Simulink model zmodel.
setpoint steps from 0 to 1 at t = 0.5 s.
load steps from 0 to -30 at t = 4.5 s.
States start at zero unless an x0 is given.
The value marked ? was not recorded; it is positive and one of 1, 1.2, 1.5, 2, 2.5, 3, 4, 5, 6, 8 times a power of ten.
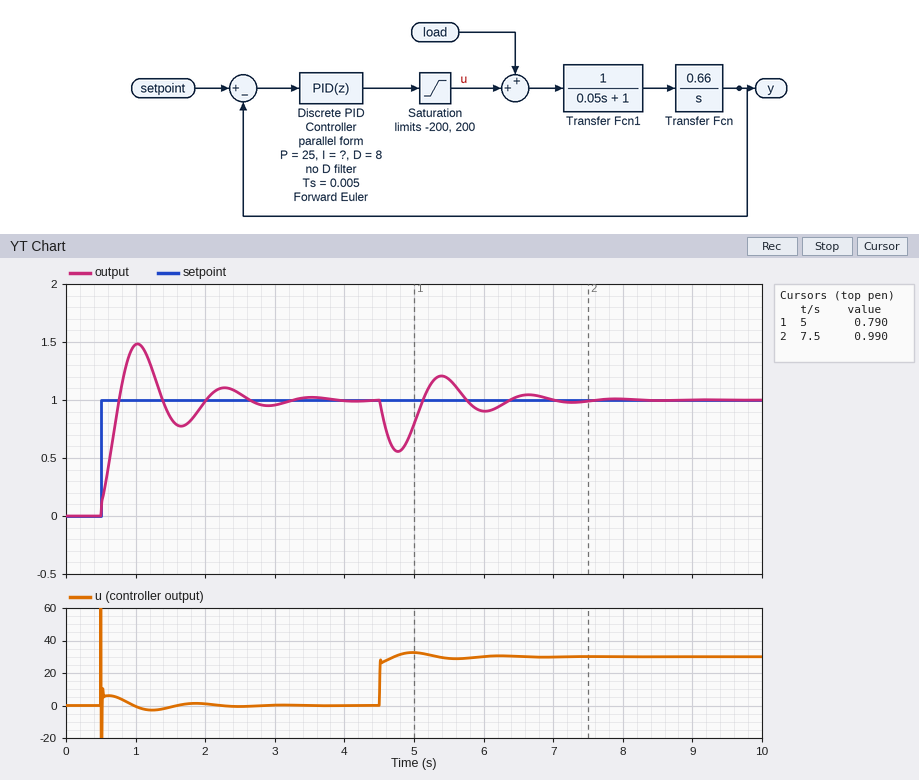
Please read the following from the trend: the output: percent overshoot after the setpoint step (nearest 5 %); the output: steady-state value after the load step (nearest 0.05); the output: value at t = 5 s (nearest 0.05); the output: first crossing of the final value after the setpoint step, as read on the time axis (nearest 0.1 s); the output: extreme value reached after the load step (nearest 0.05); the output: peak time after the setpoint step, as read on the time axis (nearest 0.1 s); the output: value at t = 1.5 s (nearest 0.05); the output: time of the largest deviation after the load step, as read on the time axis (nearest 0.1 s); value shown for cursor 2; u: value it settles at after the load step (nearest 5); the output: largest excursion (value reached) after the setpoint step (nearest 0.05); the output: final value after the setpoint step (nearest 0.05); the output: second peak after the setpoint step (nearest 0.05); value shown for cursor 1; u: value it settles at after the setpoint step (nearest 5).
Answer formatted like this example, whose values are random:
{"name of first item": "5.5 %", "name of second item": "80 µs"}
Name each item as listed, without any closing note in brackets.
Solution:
{"the output: percent overshoot after the setpoint step": "50 %", "the output: steady-state value after the load step": "1.00", "the output: value at t = 5 s": "0.80", "the output: first crossing of the final value after the setpoint step, as read on the time axis": "0.8 s", "the output: extreme value reached after the load step": "0.55", "the output: peak time after the setpoint step, as read on the time axis": "1.0 s", "the output: value at t = 1.5 s": "0.85", "the output: time of the largest deviation after the load step, as read on the time axis": "4.8 s", "value shown for cursor 2": "0.990", "u: value it settles at after the load step": "30", "the output: largest excursion (value reached) after the setpoint step": "1.50", "the output: final value after the setpoint step": "1.00", "the output: second peak after the setpoint step": "1.10", "value shown for cursor 1": "0.790", "u: value it settles at after the setpoint step": "0"}
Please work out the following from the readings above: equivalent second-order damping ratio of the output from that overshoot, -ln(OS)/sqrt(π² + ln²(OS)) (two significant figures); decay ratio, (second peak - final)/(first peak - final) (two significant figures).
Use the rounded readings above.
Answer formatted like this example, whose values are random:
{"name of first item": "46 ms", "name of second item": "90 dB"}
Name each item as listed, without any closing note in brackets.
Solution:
{"equivalent second-order damping ratio of the output from that overshoot, -ln(OS)/sqrt(π² + ln²(OS))": "0.22", "decay ratio, (second peak - final)/(first peak - final)": "0.20"}
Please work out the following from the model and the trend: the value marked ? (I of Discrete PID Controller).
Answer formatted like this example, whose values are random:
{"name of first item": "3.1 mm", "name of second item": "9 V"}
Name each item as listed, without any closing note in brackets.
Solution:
{"the value marked ?": "250"}
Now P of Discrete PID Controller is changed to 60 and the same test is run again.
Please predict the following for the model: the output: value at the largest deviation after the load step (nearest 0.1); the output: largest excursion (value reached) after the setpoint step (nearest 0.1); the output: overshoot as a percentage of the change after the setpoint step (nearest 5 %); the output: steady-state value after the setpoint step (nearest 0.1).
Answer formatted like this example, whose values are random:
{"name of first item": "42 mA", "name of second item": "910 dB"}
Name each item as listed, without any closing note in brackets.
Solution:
{"the output: value at the largest deviation after the load step": "0.7", "the output: largest excursion (value reached) after the setpoint step": "1.2", "the output: overshoot as a percentage of the change after the setpoint step": "25 %", "the output: steady-state value after the setpoint step": "1.0"}
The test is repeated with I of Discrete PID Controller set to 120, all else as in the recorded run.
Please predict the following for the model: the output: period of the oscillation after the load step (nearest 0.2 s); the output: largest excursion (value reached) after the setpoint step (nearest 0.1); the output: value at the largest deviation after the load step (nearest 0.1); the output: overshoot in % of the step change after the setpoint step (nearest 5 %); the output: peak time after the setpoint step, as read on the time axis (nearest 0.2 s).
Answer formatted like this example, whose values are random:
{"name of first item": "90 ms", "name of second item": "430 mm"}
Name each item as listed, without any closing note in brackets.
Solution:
{"the output: period of the oscillation after the load step": "1.8 s", "the output: largest excursion (value reached) after the setpoint step": "1.4", "the output: value at the largest deviation after the load step": "0.4", "the output: overshoot in % of the step change after the setpoint step": "35 %", "the output: peak time after the setpoint step, as read on the time axis": "1.2 s"}
